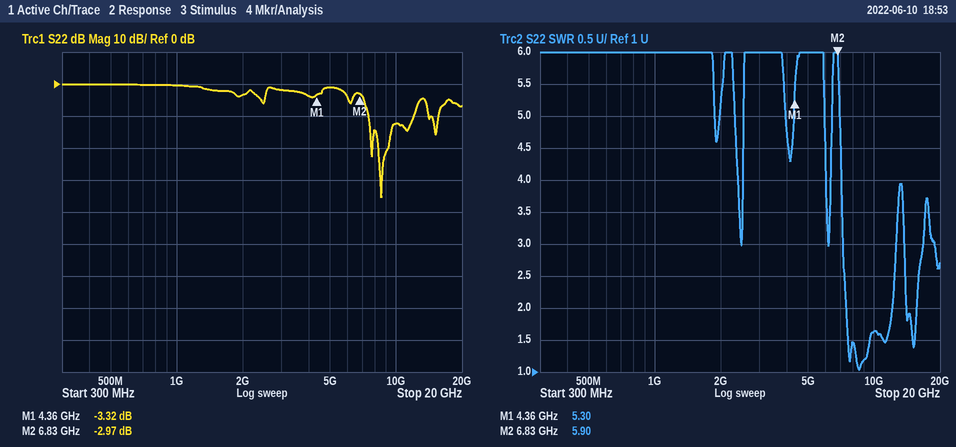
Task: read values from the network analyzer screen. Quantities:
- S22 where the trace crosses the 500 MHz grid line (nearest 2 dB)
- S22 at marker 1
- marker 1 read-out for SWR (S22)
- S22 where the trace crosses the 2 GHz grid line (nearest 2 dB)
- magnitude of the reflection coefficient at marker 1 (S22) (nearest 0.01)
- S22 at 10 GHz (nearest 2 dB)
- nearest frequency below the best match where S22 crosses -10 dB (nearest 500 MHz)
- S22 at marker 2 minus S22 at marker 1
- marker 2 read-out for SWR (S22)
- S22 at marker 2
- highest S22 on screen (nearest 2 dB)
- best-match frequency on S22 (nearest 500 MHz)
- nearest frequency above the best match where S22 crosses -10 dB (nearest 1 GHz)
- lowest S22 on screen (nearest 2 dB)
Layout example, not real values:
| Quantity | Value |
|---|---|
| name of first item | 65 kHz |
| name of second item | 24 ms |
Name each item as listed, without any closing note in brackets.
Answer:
| Quantity | Value |
|---|---|
| S22 where the trace crosses the 500 MHz grid line | 0 dB |
| S22 at marker 1 | -3.32 dB |
| marker 1 read-out for SWR | 5.30 |
| S22 where the trace crosses the 2 GHz grid line | -4 dB |
| magnitude of the reflection coefficient at marker 1 (S22) | 0.68 |
| S22 at 10 GHz | -12 dB |
| nearest frequency below the best match where S22 crosses -10 dB | 7.5 GHz |
| S22 at marker 2 minus S22 at marker 1 | 0.35 dB |
| marker 2 read-out for SWR | 5.90 |
| S22 at marker 2 | -2.97 dB |
| highest S22 on screen | 0 dB |
| best-match frequency on S22 | 8.5 GHz |
| nearest frequency above the best match where S22 crosses -10 dB | 12 GHz |
| lowest S22 on screen | -36 dB |
